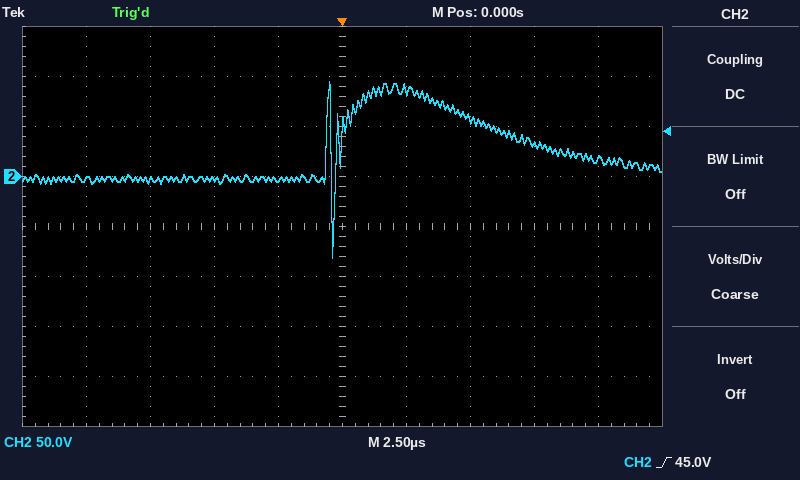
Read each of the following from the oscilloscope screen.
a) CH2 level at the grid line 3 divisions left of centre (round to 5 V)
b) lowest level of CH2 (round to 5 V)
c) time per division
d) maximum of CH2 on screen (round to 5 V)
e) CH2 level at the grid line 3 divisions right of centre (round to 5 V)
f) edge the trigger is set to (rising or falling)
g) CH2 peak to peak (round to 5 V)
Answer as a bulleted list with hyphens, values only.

- -5 V
- -80 V
- 2.5 µs
- 95 V
- 30 V
- rising
- 175 V
